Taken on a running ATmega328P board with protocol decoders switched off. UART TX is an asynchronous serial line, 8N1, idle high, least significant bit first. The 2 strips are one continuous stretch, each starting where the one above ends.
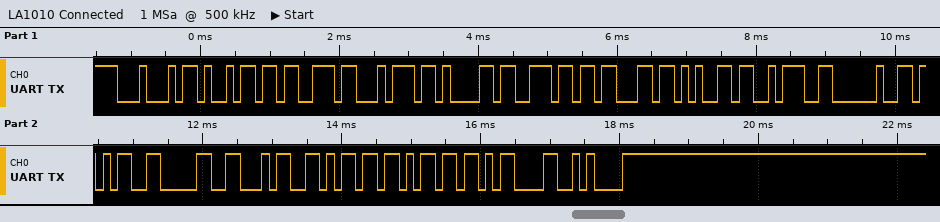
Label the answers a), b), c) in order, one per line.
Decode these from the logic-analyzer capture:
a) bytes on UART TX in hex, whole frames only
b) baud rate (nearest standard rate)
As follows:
a) 44 69 73 74 61 6E 63 65 3A 20 35 30 34 6D 6D 0D 0A
b) 9600 baud
